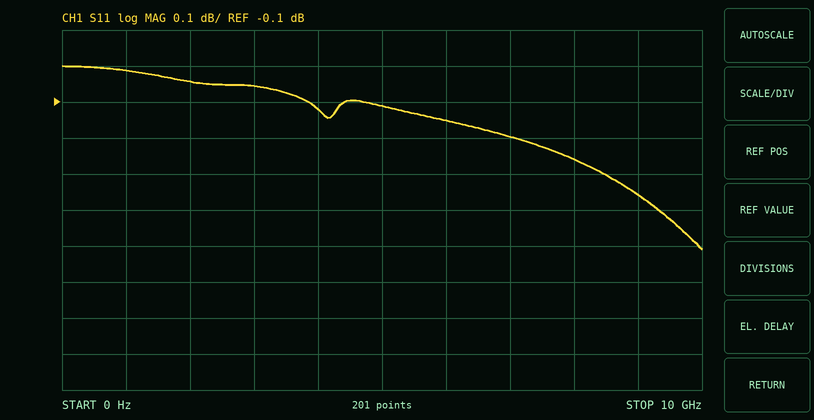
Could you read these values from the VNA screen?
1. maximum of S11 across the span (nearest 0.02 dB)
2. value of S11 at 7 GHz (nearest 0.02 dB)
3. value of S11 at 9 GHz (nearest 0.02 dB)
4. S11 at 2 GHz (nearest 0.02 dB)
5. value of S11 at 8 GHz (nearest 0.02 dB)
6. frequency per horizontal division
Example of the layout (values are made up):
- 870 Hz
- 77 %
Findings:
- 0.00 dB
- -0.20 dB
- -0.36 dB
- -0.04 dB
- -0.26 dB
- 1 GHz
